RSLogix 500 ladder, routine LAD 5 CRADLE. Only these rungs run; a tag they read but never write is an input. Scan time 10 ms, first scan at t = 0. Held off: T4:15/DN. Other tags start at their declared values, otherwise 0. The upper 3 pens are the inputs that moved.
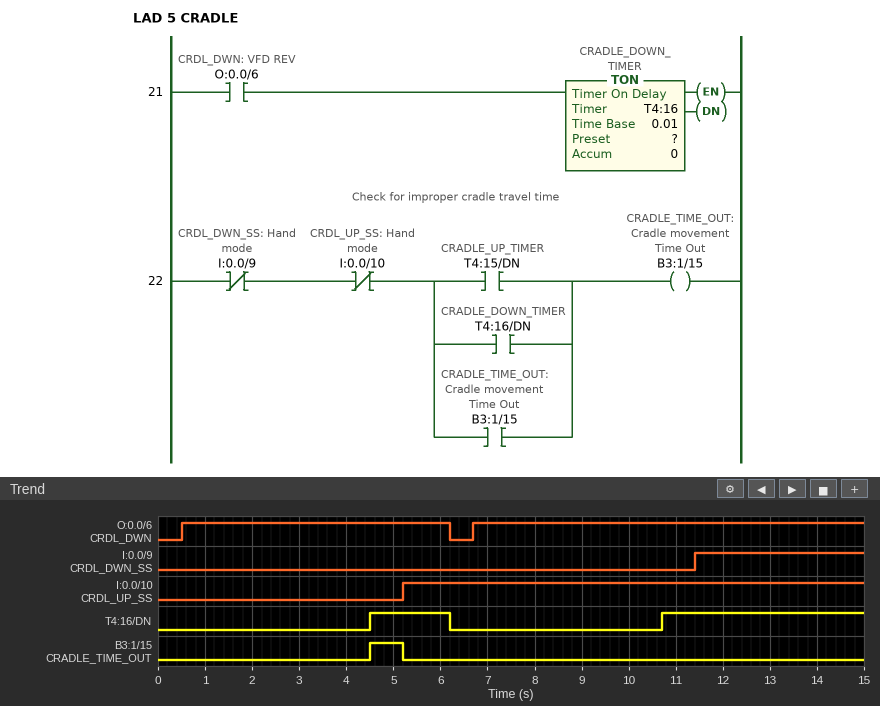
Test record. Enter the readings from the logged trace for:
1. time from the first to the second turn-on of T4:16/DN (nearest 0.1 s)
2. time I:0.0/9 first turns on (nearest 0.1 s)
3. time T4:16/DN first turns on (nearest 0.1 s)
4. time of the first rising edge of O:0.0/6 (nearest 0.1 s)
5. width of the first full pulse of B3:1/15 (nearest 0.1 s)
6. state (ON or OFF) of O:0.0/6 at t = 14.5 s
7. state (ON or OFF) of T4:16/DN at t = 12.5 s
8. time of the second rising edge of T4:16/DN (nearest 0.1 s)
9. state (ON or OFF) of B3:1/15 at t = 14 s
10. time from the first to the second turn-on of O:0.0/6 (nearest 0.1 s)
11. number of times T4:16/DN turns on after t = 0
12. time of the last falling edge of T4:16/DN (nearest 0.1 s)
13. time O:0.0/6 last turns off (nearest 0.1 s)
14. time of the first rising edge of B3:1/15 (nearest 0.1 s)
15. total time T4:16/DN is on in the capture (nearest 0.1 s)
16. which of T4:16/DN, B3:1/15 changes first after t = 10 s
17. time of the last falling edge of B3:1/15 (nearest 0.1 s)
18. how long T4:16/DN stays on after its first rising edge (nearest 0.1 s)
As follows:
6.2 s
11.4 s
4.5 s
0.5 s
0.7 s
ON
ON
10.7 s
OFF
6.2 s
2
6.2 s
6.2 s
4.5 s
6.0 s
T4:16/DN
5.2 s
1.7 s
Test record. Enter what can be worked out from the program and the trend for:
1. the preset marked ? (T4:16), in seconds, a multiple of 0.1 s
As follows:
4.0 s
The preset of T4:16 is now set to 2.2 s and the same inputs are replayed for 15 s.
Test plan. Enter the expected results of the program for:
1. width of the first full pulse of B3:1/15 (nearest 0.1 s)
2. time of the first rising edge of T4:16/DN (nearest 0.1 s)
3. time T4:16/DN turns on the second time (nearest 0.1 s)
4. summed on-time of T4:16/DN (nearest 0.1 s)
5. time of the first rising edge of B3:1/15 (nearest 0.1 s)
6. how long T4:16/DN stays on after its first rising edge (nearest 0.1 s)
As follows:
2.5 s
2.7 s
8.9 s
9.6 s
2.7 s
3.5 s
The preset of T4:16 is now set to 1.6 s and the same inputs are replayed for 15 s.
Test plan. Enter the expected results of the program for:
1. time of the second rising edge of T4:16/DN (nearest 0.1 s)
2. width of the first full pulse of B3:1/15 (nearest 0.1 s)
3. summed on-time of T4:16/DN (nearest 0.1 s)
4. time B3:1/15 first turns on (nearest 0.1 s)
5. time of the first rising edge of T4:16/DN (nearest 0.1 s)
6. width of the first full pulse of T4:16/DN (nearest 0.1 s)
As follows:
8.3 s
3.1 s
10.8 s
2.1 s
2.1 s
4.1 s
